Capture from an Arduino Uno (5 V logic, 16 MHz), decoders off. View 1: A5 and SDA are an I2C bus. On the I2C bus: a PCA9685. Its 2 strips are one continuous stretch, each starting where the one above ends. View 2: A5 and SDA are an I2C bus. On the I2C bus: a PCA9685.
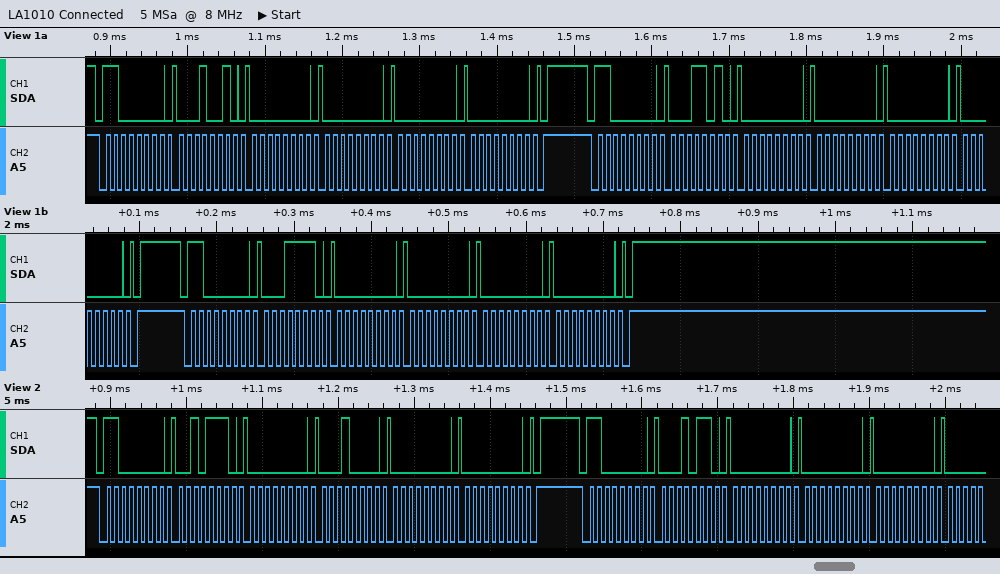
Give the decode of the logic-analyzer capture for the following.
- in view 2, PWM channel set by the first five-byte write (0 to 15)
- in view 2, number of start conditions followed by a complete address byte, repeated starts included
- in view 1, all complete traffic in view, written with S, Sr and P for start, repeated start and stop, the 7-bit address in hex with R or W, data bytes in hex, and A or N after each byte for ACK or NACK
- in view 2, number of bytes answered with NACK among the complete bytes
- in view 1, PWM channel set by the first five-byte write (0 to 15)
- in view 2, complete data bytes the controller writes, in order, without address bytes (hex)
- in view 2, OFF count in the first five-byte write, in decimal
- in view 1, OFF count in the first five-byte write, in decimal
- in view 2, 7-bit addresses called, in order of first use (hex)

10
2
S 60W A 12 A 00 A 00 A 00 A 00 A P S 60W A 1A A 00 A 00 A 00 A 00 A P S 60W A 1E A 00 A 00 A 00 A 00 A P
0
3
2E 00 10 00 00 16 00 00 00
0
0
0x60
